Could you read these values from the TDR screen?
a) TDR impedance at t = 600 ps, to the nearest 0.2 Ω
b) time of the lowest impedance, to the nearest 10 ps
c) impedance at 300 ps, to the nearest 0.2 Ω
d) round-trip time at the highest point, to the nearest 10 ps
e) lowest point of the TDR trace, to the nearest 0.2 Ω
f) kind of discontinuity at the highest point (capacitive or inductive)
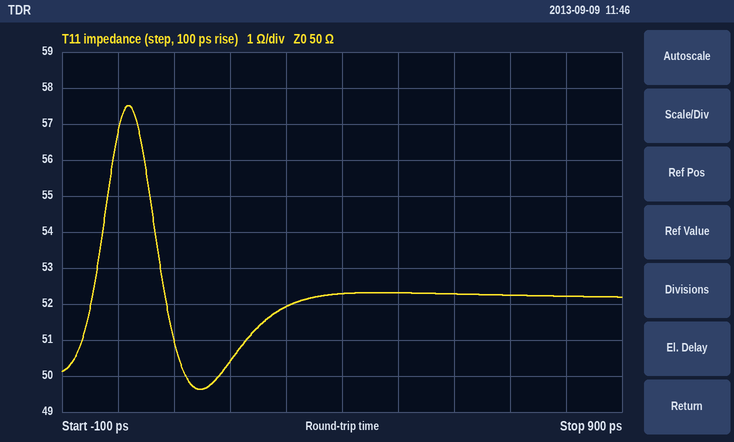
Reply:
52.2 Ω
150 ps
52.0 Ω
20 ps
49.6 Ω
inductive
